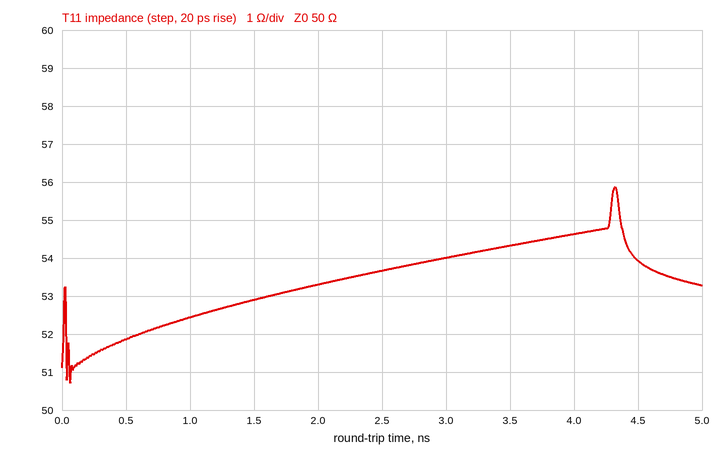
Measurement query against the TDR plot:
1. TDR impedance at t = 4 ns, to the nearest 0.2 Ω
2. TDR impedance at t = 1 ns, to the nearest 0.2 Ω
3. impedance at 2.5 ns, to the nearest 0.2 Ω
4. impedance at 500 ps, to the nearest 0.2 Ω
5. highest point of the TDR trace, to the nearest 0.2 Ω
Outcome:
54.6 Ω
52.4 Ω
53.6 Ω
51.8 Ω
55.8 Ω
